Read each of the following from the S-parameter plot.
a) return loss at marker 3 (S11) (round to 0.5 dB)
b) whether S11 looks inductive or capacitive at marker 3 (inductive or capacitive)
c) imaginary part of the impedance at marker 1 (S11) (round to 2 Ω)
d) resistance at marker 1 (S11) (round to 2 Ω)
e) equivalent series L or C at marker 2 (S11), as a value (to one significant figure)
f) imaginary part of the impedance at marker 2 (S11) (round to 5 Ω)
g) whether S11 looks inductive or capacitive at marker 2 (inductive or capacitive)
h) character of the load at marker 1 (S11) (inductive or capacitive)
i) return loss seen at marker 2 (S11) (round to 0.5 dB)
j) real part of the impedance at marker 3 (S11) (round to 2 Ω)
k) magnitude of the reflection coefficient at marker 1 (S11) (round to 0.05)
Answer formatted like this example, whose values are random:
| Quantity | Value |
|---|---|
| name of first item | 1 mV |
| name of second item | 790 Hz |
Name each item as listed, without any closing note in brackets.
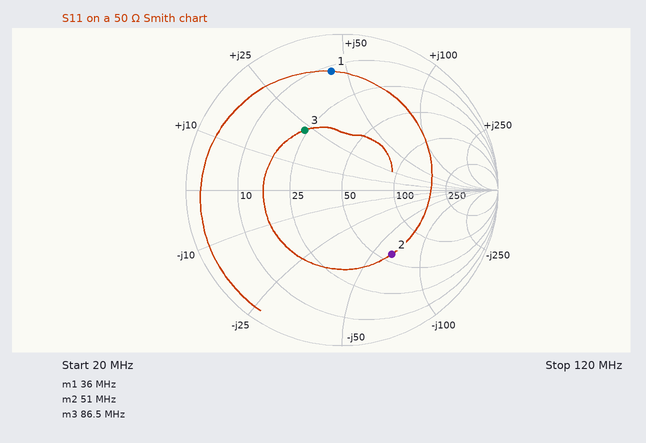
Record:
| Quantity | Value |
|---|---|
| return loss at marker 3 (S11) | 7.0 dB |
| whether S11 looks inductive or capacitive at marker 3 | inductive |
| imaginary part of the impedance at marker 1 (S11) | +44 Ω |
| resistance at marker 1 (S11) | 12 Ω |
| equivalent series L or C at marker 2 (S11), as a value | 50 pF |
| imaginary part of the impedance at marker 2 (S11) | -65 Ω |
| whether S11 looks inductive or capacitive at marker 2 | capacitive |
| character of the load at marker 1 (S11) | inductive |
| return loss seen at marker 2 (S11) | 5.5 dB |
| real part of the impedance at marker 3 (S11) | 24 Ω |
| magnitude of the reflection coefficient at marker 1 (S11) | 0.75 |
